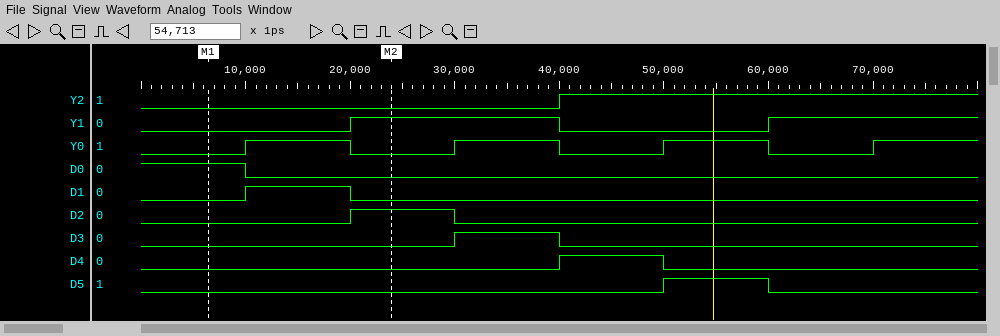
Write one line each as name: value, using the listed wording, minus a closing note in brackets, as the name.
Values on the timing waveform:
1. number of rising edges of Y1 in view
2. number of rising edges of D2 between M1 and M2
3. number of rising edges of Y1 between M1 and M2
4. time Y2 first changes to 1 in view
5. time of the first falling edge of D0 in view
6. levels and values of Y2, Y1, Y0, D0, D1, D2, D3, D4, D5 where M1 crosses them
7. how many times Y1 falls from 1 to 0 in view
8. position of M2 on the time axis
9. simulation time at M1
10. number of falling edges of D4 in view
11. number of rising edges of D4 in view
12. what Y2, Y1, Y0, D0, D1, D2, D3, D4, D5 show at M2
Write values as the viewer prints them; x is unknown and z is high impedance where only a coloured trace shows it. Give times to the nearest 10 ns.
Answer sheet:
number of rising edges of Y1 in view: 2
number of rising edges of D2 between M1 and M2: 1
number of rising edges of Y1 between M1 and M2: 1
time Y2 first changes to 1 in view: 40 ns
time of the first falling edge of D0 in view: 10 ns
levels and values of Y2, Y1, Y0, D0, D1, D2, D3, D4, D5 where M1 crosses them: Y2=0, Y1=0, Y0=0, D0=1, D1=0, D2=0, D3=0, D4=0, D5=0
how many times Y1 falls from 1 to 0 in view: 1
position of M2 on the time axis: 20 ns
simulation time at M1: 10 ns
number of falling edges of D4 in view: 1
number of rising edges of D4 in view: 1
what Y2, Y1, Y0, D0, D1, D2, D3, D4, D5 show at M2: Y2=0, Y1=1, Y0=0, D0=0, D1=0, D2=1, D3=0, D4=0, D5=0
